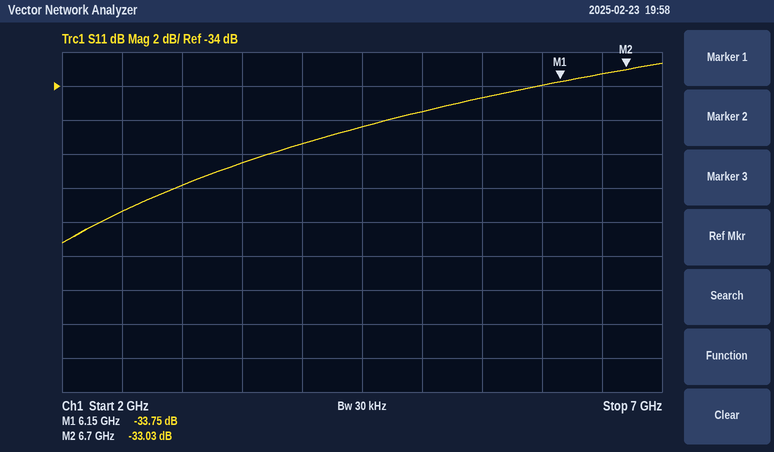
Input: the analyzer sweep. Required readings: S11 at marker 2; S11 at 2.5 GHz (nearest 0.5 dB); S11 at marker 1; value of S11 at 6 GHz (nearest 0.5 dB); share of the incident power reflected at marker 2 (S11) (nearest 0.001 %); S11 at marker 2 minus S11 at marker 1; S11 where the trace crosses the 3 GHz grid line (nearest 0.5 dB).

-33.03 dB
-41.5 dB
-33.75 dB
-34.0 dB
0.050 %
0.72 dB
-40.0 dB
